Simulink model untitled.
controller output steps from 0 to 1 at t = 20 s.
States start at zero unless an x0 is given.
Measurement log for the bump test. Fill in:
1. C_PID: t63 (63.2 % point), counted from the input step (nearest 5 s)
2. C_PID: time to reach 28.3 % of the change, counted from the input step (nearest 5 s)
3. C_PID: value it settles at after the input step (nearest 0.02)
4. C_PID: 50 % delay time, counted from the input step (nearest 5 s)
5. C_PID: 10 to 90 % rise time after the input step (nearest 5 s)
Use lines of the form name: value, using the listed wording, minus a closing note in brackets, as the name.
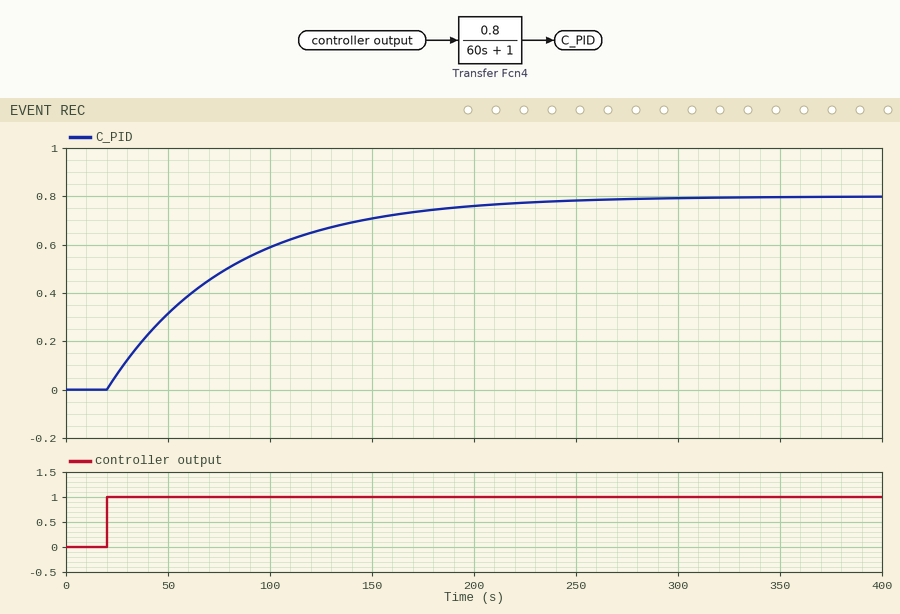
C_PID: t63 (63.2 % point), counted from the input step: 60 s
C_PID: time to reach 28.3 % of the change, counted from the input step: 20 s
C_PID: value it settles at after the input step: 0.80
C_PID: 50 % delay time, counted from the input step: 40 s
C_PID: 10 to 90 % rise time after the input step: 130 s
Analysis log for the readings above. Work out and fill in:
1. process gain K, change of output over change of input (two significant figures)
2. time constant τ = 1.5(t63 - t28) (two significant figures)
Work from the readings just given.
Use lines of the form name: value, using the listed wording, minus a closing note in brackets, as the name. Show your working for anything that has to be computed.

process gain K, change of output over change of input: (0.8 - 0) / 1 = 0.80
time constant τ = 1.5(t63 - t28): 1.5 × (60 - 20) = 60 s
